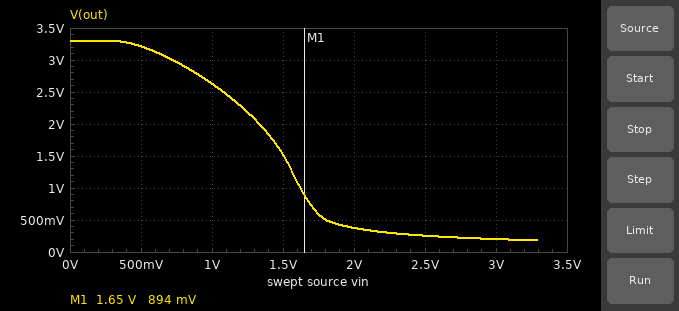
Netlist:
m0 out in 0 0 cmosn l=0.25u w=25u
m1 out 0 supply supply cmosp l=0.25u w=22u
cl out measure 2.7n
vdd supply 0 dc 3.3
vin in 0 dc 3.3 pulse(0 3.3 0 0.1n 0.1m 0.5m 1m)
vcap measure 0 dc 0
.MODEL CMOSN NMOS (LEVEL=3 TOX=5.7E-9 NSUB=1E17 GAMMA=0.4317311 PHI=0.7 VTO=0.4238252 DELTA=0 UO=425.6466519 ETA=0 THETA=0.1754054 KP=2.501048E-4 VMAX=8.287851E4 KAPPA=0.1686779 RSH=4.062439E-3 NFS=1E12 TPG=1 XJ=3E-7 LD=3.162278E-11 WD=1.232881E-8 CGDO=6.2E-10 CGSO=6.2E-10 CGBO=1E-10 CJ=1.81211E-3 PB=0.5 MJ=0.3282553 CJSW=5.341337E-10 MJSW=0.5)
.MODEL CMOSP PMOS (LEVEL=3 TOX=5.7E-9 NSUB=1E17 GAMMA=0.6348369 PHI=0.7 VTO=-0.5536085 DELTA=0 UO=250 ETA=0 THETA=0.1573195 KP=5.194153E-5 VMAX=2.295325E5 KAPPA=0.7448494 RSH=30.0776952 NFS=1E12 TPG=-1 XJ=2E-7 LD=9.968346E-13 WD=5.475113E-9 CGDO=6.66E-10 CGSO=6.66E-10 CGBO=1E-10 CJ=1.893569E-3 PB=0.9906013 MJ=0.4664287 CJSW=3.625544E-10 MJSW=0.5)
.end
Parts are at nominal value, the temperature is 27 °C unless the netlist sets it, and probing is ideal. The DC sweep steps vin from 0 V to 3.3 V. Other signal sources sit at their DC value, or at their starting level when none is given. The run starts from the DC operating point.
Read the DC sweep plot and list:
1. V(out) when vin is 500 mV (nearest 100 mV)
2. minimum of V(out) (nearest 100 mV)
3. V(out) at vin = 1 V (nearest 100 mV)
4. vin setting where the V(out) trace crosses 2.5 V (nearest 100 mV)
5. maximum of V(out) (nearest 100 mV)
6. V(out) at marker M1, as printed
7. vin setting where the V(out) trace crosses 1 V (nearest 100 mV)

3.2 V
200 mV
2.6 V
1.1 V
3.3 V
894 mV
1.6 V
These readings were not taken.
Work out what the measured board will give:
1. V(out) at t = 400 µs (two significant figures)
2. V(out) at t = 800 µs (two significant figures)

180 mV
3.3 V
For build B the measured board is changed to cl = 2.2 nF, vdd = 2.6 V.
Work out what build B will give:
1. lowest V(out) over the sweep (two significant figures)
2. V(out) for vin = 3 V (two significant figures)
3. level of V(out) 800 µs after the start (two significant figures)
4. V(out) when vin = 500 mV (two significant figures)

110 mV
120 mV
2.6 V
2.5 V
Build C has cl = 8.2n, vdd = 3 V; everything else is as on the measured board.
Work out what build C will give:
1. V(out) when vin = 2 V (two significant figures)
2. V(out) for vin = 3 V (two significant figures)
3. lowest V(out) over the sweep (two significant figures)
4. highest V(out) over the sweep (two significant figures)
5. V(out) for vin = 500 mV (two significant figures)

280 mV
160 mV
150 mV
3.0 V
2.9 V
